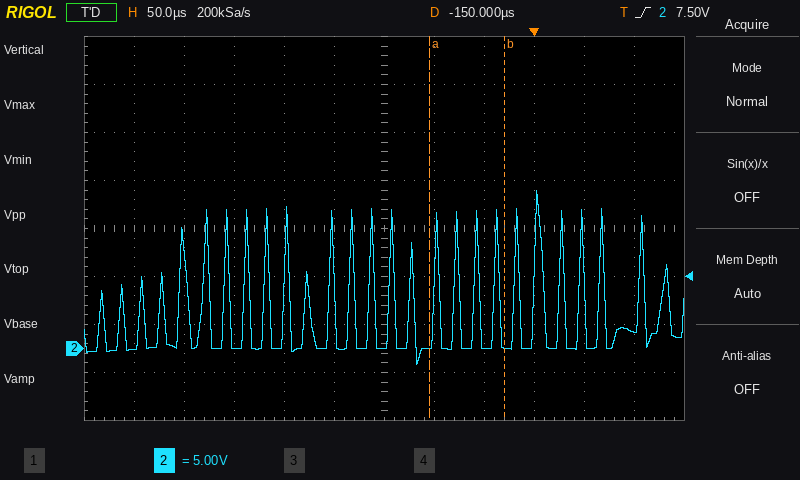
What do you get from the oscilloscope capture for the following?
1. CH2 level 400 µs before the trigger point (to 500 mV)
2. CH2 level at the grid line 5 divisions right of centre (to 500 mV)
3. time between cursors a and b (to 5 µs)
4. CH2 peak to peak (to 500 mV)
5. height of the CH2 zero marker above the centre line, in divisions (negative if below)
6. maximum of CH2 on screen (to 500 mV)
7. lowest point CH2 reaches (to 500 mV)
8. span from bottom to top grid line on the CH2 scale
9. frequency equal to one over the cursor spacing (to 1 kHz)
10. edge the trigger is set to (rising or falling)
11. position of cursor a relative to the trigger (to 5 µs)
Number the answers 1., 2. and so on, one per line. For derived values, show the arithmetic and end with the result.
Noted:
1. 0.0 V
2. 2.0 V
3. 75 µs
4. 16.5 V − (-1.5 V) = 18.0 V
5. -2.5 div
6. 16.5 V
7. -1.5 V
8. 40 V
9. 1 / 75 µs ≈ 13 kHz
10. rising
11. -105 µs
